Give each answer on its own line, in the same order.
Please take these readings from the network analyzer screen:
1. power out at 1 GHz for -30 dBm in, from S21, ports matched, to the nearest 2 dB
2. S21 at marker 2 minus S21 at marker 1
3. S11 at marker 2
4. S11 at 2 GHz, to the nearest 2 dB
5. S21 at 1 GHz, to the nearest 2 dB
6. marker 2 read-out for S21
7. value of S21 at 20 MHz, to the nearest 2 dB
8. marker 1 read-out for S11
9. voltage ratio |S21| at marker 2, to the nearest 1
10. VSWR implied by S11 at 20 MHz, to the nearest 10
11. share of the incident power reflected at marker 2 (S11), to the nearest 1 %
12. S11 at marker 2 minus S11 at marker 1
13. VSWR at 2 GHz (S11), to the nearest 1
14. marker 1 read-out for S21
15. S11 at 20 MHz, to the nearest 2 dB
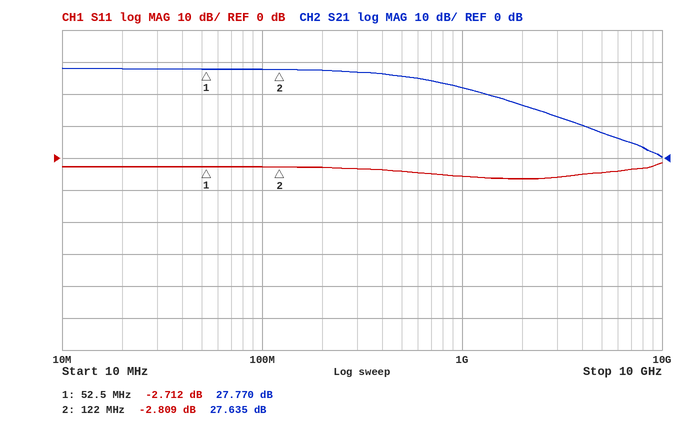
-8 dBm
-0.135 dB
-2.809 dB
-6 dB
22 dB
27.635 dB
28 dB
-2.712 dB
24
10
52 %
-0.097 dB
3
27.770 dB
-2 dB
